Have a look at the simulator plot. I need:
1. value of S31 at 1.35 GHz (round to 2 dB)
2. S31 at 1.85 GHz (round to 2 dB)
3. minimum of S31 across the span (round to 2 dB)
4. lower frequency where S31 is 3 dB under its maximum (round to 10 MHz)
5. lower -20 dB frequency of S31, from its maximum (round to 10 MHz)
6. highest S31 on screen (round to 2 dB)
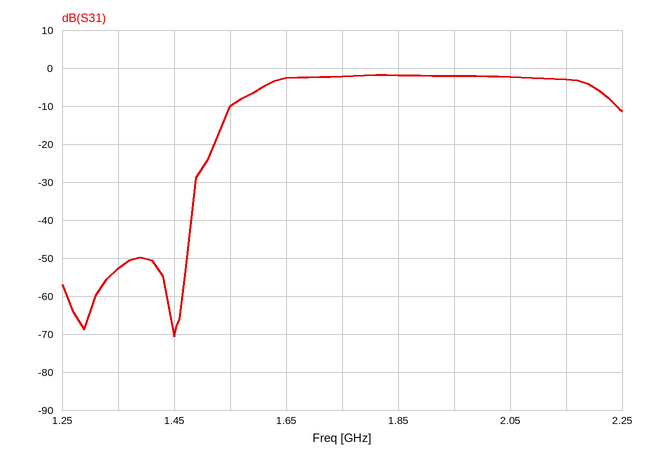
-52 dB
-2 dB
-70 dB
1.61 GHz
1.52 GHz
-2 dB
